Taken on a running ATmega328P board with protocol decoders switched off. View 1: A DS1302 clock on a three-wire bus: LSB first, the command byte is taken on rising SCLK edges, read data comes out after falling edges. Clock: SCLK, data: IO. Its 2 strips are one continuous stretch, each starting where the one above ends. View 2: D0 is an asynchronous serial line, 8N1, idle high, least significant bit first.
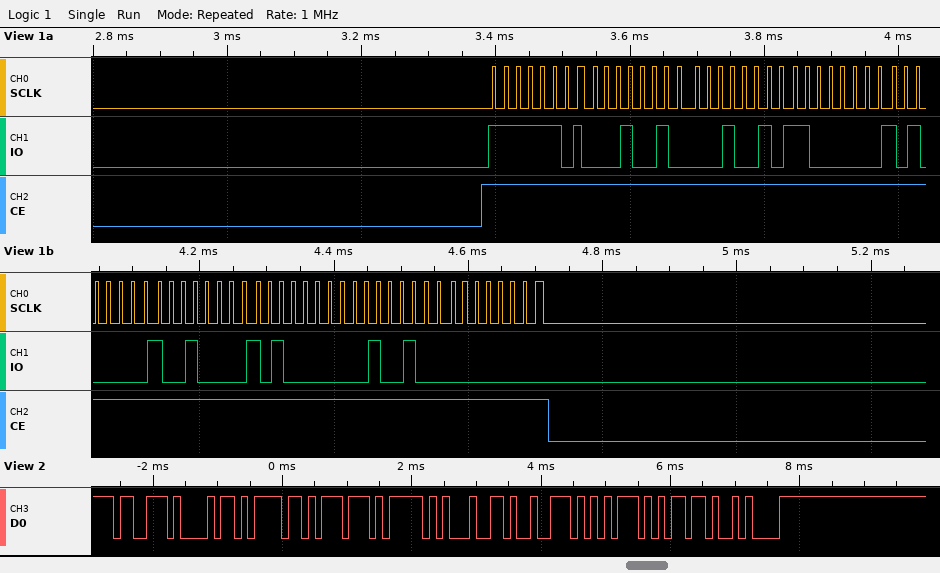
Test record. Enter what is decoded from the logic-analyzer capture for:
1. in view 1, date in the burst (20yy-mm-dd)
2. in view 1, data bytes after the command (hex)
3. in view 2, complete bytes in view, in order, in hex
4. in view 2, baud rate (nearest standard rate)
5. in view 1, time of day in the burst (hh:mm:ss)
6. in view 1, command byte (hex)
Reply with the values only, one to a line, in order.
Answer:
2024-09-05
48 48 03 05 09 05 24 00
0x73 0x68 0x6F 0x77 0x5F 0x64 0x72 0x75 0x6D 0x0A
9600 baud
03:48:48
0xBF
